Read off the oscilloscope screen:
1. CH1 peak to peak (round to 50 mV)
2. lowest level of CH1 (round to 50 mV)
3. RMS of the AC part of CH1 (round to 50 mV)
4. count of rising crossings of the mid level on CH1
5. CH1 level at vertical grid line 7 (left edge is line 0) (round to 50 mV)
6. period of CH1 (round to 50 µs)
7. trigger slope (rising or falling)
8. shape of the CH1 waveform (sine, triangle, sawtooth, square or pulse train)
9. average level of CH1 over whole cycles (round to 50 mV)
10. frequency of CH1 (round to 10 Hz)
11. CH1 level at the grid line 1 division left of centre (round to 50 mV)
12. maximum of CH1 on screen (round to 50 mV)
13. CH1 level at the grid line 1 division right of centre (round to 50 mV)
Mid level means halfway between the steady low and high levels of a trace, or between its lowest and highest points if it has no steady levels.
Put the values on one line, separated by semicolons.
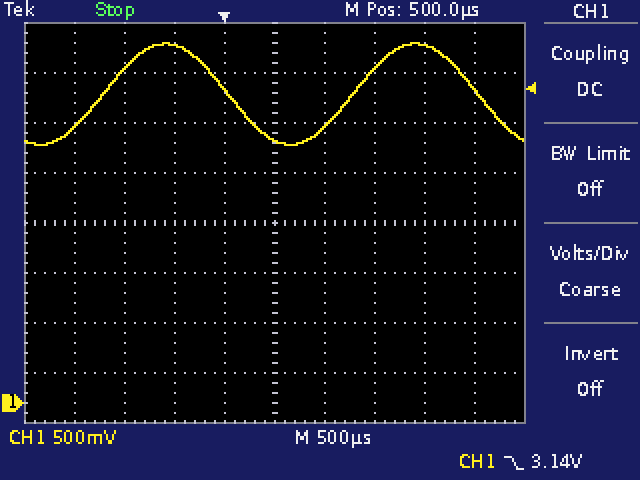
1.00 V; 2.60 V; 350 mV; 2; 3.35 V; 2.50 ms; falling; sine; 3.10 V; 400 Hz; 3.15 V; 3.60 V; 2.75 V
